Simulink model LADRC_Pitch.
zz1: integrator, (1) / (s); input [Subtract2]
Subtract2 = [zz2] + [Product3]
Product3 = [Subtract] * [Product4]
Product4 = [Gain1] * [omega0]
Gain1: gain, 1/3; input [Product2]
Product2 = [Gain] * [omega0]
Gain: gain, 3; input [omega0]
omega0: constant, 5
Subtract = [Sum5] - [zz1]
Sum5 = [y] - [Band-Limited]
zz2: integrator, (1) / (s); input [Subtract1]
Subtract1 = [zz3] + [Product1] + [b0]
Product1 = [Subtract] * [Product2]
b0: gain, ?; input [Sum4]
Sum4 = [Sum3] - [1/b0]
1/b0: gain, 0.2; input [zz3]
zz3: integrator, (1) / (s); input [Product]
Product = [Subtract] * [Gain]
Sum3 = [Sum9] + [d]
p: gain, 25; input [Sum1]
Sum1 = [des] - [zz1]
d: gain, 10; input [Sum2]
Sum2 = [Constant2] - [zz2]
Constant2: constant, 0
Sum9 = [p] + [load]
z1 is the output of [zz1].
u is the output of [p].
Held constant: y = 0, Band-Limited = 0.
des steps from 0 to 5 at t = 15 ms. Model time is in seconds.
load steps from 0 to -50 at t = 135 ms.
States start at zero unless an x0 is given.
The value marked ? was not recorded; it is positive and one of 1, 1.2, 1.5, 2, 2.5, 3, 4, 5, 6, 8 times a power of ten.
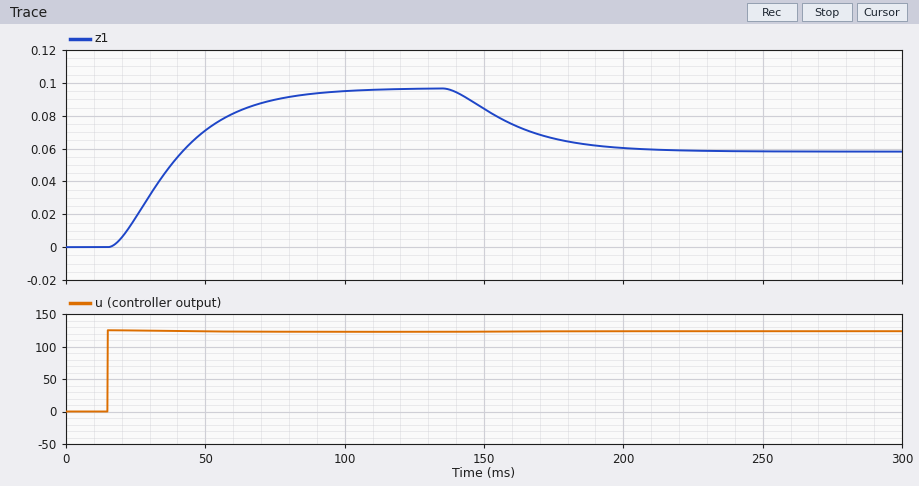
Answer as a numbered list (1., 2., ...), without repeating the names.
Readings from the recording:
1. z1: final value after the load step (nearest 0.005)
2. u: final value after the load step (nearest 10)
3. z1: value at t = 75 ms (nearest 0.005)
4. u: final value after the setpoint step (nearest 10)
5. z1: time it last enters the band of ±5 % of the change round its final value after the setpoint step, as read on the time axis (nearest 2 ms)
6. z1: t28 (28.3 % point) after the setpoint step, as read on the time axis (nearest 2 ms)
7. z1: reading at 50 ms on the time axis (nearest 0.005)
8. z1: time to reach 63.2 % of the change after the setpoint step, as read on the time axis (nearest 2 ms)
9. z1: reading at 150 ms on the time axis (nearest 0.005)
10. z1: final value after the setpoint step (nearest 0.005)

1. 0.060
2. 120
3. 0.090
4. 120
5. 82 ms
6. 28 ms
7. 0.070
8. 44 ms
9. 0.085
10. 0.095
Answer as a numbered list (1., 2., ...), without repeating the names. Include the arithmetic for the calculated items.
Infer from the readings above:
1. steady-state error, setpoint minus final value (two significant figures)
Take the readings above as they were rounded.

1. 5 - 0.095 = 4.9
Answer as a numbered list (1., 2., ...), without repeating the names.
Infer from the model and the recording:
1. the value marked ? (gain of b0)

1. 5
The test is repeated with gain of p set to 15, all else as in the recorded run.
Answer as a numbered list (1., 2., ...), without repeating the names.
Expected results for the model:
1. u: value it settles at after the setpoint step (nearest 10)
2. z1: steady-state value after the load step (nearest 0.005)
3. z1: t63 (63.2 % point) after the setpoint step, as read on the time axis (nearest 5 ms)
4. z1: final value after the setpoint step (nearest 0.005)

1. 70
2. 0.020
3. 45 ms
4. 0.060
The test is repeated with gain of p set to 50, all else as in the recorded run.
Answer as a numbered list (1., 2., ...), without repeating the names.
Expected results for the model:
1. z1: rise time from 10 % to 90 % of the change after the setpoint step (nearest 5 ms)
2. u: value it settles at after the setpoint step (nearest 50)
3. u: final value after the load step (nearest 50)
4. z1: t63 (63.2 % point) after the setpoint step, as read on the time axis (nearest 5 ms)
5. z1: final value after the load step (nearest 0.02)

1. 45 ms
2. 250
3. 250
4. 45 ms
5. 0.16
